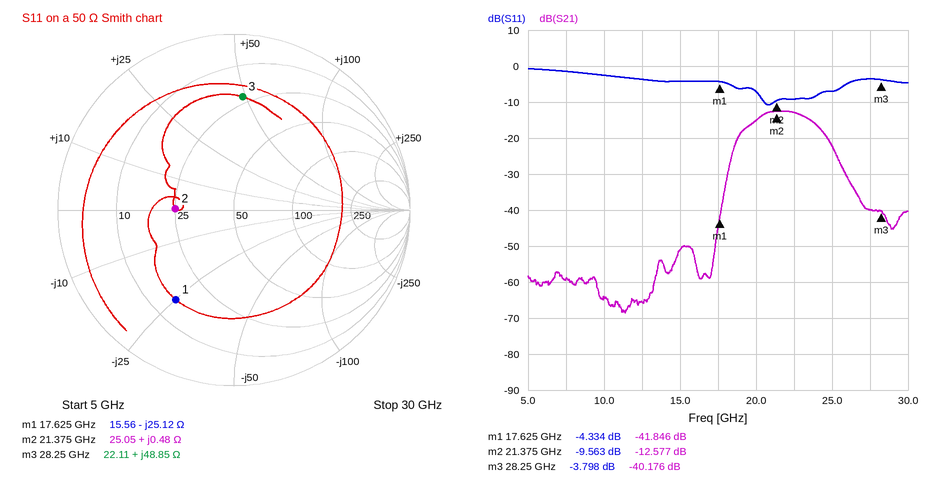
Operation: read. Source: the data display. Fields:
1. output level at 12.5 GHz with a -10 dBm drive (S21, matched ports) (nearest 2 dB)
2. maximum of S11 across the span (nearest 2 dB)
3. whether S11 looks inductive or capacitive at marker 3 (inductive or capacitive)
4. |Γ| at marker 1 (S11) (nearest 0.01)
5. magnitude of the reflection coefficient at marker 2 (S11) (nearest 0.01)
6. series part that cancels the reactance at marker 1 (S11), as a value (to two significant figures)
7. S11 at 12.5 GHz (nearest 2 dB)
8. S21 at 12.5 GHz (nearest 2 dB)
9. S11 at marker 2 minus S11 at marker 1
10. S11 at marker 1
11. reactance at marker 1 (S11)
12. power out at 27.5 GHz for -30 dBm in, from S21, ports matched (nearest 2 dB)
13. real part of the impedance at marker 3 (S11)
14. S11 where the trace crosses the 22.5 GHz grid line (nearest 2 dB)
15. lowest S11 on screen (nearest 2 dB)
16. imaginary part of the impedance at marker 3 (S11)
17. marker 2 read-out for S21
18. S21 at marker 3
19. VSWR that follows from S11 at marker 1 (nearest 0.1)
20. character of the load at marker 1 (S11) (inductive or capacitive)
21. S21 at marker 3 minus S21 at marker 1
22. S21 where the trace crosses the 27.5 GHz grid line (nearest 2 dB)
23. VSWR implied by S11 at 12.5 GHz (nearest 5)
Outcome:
-76 dBm
0 dB
inductive
0.61
0.33
230 pH
-4 dB
-66 dB
-5.229 dB
-4.334 dB
-25.12 Ω
-70 dBm
22.11 Ω
-10 dB
-10 dB
+48.85 Ω
-12.577 dB
-40.176 dB
4.1
capacitive
1.670 dB
-40 dB
5
